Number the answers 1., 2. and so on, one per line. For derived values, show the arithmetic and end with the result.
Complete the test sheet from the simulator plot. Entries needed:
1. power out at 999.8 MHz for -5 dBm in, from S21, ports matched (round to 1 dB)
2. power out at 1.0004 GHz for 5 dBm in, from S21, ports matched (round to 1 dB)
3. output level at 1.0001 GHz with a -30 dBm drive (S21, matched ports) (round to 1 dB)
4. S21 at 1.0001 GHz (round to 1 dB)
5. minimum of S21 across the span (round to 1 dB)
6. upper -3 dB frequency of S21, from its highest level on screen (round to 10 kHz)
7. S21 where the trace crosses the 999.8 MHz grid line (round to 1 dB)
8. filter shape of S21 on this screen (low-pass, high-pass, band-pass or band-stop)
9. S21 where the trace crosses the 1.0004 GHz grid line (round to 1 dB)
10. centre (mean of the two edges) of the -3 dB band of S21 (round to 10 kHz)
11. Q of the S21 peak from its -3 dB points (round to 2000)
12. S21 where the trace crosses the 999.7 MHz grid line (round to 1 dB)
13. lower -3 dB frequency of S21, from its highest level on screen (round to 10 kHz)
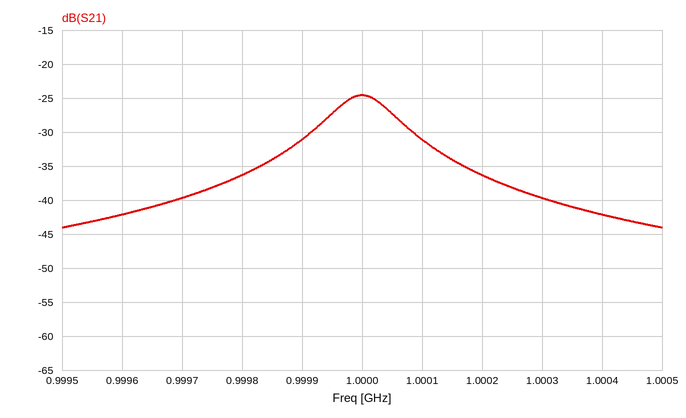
1. -5 dBm + (-36 dB) = -41 dBm
2. 5 dBm + (-42 dB) = -37 dBm
3. -30 dBm + (-31 dB) = -61 dBm
4. -31 dB
5. -44 dB
6. 1.00005 GHz
7. -36 dB
8. band-pass
9. -42 dB
10. 1.00000 GHz
11. 1 GHz / 100 kHz ≈ 10000
12. -40 dB
13. 999.95 MHz
